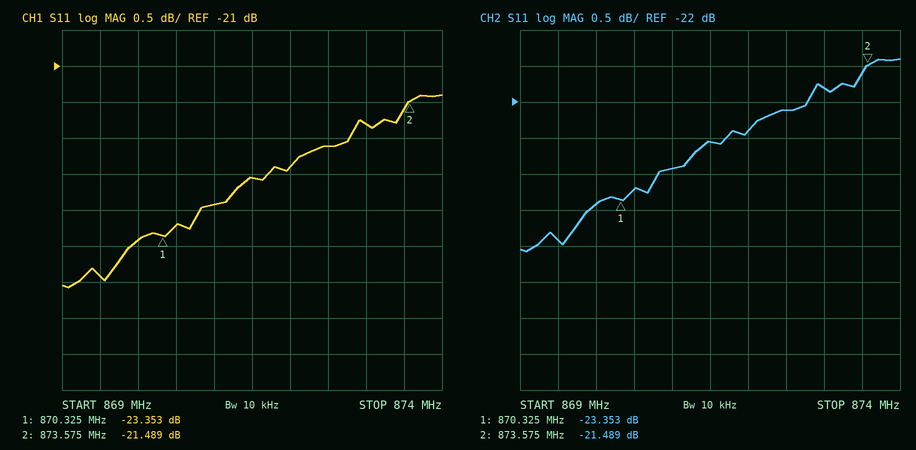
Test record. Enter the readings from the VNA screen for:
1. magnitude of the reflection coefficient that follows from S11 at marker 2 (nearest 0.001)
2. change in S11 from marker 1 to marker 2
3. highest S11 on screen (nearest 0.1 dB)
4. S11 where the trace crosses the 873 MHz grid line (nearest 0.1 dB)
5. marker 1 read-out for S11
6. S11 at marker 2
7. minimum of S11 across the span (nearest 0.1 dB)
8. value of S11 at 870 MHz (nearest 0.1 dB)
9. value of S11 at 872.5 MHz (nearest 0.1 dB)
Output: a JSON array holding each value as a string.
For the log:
["0.084", "1.864 dB", "-21.4 dB", "-21.8 dB", "-23.353 dB", "-21.489 dB", "-24.1 dB", "-23.4 dB", "-22.1 dB"]
